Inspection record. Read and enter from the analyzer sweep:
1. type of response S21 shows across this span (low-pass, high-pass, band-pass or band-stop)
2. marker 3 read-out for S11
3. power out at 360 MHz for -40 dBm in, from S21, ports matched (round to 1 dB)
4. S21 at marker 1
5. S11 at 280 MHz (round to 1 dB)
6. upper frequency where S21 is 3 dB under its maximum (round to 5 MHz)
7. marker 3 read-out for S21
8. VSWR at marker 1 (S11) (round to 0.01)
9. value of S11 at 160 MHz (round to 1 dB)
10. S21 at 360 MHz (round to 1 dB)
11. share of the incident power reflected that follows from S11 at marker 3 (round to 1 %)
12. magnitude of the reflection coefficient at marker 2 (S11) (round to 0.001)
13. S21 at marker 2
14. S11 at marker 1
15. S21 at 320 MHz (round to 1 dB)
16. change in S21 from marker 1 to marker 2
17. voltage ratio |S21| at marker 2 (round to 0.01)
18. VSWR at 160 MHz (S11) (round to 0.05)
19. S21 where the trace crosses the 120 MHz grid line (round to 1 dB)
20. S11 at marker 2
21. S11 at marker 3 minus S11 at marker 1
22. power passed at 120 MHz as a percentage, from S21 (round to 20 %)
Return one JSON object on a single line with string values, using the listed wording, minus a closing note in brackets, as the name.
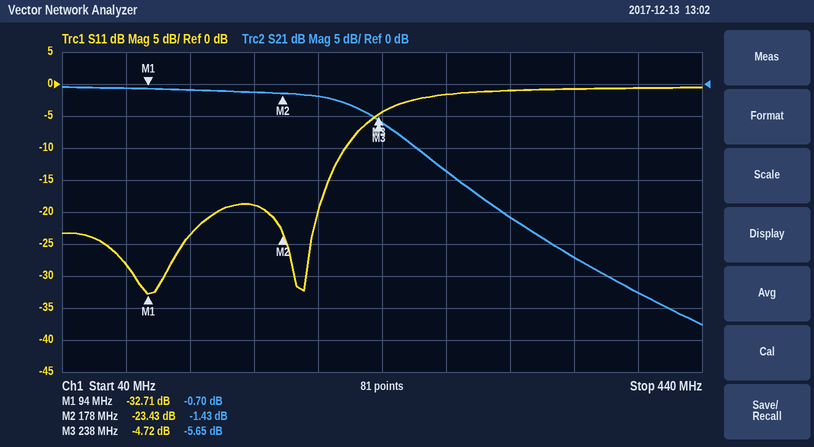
{"type of response S21 shows across this span": "low-pass", "marker 3 read-out for S11": "-4.72 dB", "power out at 360 MHz for -40 dBm in, from S21, ports matched": "-67 dBm", "S21 at marker 1": "-0.70 dB", "S11 at 280 MHz": "-2 dB", "upper frequency where S21 is 3 dB under its maximum": "220 MHz", "marker 3 read-out for S21": "-5.65 dB", "VSWR at marker 1 (S11)": "1.05", "value of S11 at 160 MHz": "-19 dB", "S21 at 360 MHz": "-27 dB", "share of the incident power reflected that follows from S11 at marker 3": "34 %", "magnitude of the reflection coefficient at marker 2 (S11)": "0.067", "S21 at marker 2": "-1.43 dB", "S11 at marker 1": "-32.71 dB", "S21 at 320 MHz": "-21 dB", "change in S21 from marker 1 to marker 2": "-0.73 dB", "voltage ratio |S21| at marker 2": "0.85", "VSWR at 160 MHz (S11)": "1.25", "S21 where the trace crosses the 120 MHz grid line": "-1 dB", "S11 at marker 2": "-23.43 dB", "S11 at marker 3 minus S11 at marker 1": "27.99 dB", "power passed at 120 MHz as a percentage, from S21": "80 %"}
